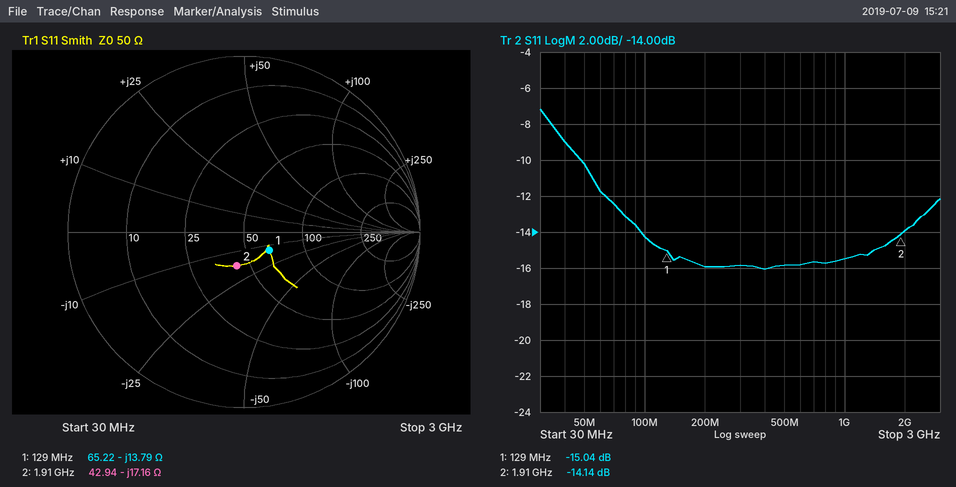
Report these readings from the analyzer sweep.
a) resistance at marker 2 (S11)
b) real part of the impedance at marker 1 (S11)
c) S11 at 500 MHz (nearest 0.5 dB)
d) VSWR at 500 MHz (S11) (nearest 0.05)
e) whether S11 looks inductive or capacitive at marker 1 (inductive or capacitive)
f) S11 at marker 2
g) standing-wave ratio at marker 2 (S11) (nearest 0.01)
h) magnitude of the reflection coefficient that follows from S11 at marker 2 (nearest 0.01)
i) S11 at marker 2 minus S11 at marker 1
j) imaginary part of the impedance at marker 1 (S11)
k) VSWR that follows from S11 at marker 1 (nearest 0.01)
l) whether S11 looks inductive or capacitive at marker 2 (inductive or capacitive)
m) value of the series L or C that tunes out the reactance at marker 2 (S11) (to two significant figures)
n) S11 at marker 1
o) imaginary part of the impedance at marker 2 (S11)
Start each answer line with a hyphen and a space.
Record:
- 42.94 Ω
- 65.22 Ω
- -16.0 dB
- 1.40
- capacitive
- -14.14 dB
- 1.49
- 0.20
- 0.90 dB
- -13.79 Ω
- 1.43
- capacitive
- 1.4 nH
- -15.04 dB
- -17.16 Ω
